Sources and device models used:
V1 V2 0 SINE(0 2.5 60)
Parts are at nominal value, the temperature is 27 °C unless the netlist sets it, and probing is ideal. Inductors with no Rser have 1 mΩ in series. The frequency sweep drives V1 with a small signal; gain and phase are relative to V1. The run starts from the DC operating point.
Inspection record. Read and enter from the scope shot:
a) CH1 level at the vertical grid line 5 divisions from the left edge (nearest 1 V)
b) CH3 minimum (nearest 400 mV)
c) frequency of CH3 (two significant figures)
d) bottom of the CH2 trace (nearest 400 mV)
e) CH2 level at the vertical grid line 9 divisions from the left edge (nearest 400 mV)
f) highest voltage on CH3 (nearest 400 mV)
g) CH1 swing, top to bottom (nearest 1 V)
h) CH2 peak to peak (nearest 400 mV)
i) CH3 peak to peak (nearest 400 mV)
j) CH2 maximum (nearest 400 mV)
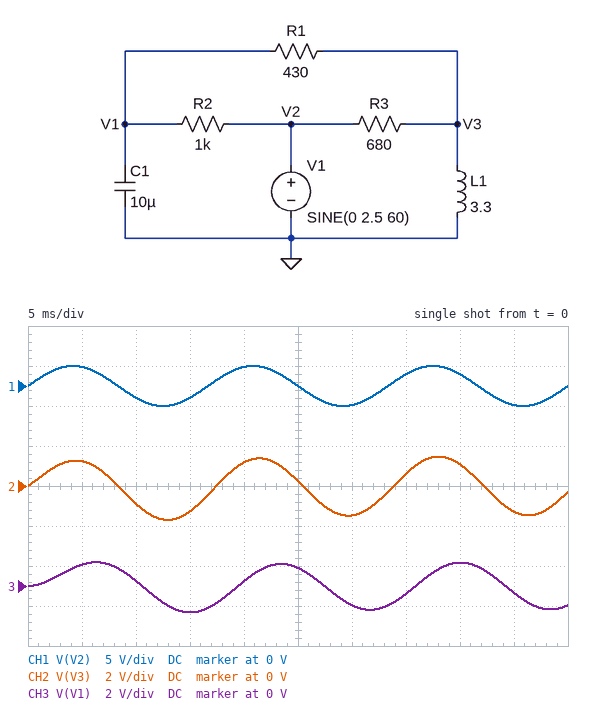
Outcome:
0 V
-1.2 V
61 Hz
-1.6 V
-1.2 V
1.2 V
5 V
3.2 V
2.4 V
1.6 V
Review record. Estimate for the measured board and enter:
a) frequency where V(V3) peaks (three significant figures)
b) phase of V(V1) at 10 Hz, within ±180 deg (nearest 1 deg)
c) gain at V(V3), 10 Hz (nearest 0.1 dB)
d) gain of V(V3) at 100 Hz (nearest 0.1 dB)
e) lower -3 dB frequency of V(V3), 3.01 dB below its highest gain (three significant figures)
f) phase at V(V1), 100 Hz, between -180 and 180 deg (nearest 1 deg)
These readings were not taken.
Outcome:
28.1 Hz
19 deg
-7.4 dB
-6.4 dB
12.9 Hz
-69 deg
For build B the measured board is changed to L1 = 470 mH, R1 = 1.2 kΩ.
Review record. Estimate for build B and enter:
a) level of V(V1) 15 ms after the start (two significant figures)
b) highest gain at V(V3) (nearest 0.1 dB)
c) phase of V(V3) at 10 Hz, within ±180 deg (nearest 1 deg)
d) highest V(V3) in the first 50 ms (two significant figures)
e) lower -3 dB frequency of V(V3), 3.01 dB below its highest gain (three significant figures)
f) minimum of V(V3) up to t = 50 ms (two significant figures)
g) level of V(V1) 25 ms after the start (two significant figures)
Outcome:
-640 mV
-3.9 dB
82 deg
660 mV
137 Hz
-670 mV
550 mV
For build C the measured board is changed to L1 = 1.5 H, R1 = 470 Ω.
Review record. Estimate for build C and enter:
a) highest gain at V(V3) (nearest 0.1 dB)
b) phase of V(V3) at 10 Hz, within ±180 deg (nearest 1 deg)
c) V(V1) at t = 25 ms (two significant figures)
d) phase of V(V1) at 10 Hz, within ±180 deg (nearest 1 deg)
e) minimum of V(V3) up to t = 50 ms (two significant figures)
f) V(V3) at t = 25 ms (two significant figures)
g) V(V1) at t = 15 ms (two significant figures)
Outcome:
-4.8 dB
74 deg
800 mV
9 deg
-1.5 V
-200 mV
-1.2 V
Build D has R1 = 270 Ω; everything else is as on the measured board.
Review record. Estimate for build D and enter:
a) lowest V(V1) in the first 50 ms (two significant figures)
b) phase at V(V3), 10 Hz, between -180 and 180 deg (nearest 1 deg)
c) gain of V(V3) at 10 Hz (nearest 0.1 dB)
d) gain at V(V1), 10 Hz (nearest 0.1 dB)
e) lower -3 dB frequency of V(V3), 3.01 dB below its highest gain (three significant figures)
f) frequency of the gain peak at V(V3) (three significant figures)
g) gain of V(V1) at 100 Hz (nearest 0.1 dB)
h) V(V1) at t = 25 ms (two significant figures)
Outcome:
-1.5 V
60 deg
-7.0 dB
-6.2 dB
13.1 Hz
27.3 Hz
-9.9 dB
960 mV
